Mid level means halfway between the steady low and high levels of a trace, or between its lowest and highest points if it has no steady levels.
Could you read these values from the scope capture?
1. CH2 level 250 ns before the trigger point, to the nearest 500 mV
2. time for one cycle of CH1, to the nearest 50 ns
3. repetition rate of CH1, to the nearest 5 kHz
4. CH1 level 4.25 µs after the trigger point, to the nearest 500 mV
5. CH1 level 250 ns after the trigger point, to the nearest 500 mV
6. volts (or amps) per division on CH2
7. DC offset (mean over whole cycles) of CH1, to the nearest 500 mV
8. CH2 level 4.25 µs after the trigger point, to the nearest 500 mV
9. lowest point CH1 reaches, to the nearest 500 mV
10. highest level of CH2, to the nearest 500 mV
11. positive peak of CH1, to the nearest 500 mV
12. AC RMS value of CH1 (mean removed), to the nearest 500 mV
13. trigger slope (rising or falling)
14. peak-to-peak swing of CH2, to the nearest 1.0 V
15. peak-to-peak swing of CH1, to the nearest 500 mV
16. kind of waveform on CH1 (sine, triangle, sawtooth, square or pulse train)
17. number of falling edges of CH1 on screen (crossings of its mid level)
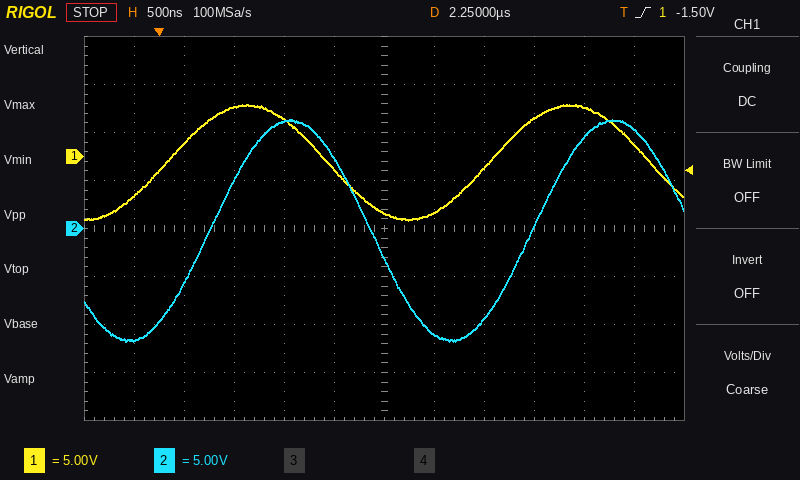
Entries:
-11.5 V
3.25 µs
310 kHz
5.0 V
1.5 V
5 V
-500 mV
9.5 V
-6.5 V
11.5 V
5.5 V
4.0 V
rising
23.0 V
12.0 V
sine
2
